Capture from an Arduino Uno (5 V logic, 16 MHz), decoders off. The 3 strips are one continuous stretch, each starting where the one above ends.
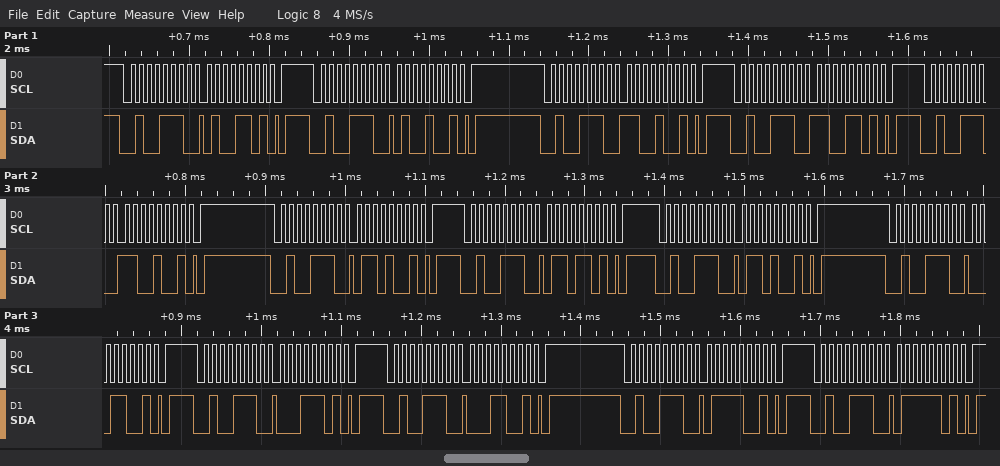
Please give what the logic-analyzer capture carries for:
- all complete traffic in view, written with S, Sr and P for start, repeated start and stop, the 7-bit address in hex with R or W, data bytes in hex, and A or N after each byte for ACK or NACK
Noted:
S 27W A 4D A P S 27W A 49 A P S 27W A C9 A P S 27W A CD A P S 27W A C9 A P S 27W A 69 A P S 27W A 6D A P S 27W A 69 A P S 27W A 19 A P S 27W A 1D A P S 27W A 19 A P S 27W A 79 A P S 27W A 7D A P
